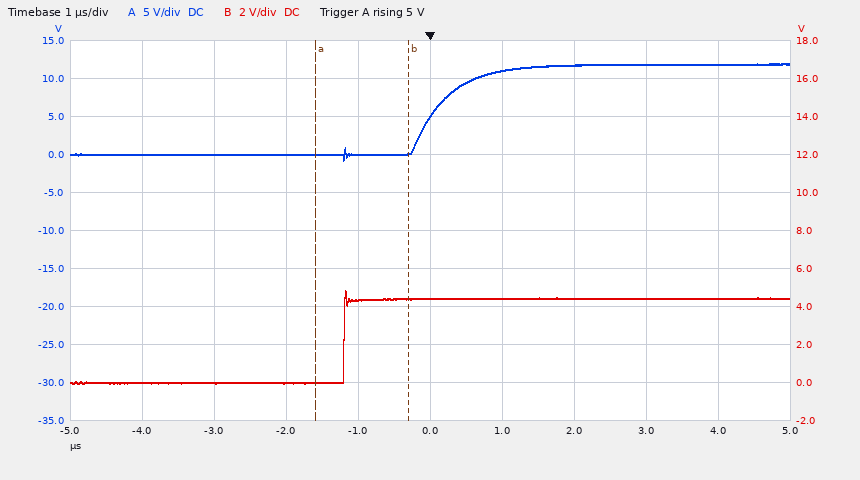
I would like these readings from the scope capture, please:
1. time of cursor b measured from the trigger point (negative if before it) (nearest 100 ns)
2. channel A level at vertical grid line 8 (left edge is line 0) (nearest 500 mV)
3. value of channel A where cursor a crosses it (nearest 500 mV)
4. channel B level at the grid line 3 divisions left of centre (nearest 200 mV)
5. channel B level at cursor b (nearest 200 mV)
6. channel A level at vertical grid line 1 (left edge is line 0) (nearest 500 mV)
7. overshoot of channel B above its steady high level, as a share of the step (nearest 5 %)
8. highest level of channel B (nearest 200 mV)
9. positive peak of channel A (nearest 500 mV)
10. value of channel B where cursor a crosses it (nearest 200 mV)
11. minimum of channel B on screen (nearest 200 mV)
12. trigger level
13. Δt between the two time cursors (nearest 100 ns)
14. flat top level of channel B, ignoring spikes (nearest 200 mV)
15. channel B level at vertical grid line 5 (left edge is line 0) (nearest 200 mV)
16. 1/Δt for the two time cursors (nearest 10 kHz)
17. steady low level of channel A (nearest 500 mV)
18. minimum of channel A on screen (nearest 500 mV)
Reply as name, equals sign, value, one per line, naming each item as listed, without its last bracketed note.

time of cursor b measured from the trigger point (negative if before it) = -300 ns
channel A level at vertical grid line 8 (left edge is line 0) = 12.0 V
value of channel A where cursor a crosses it = 0.0 V
channel B level at the grid line 3 divisions left of centre = 0.0 V
channel B level at cursor b = 4.4 V
channel A level at vertical grid line 1 (left edge is line 0) = 0.0 V
overshoot of channel B above its steady high level, as a share of the step = 10 %
highest level of channel B = 4.8 V
positive peak of channel A = 12.0 V
value of channel B where cursor a crosses it = 0.0 V
minimum of channel B on screen = 0.0 V
trigger level = 5 V
Δt between the two time cursors = 1.3 µs
flat top level of channel B, ignoring spikes = 4.4 V
channel B level at vertical grid line 5 (left edge is line 0) = 4.4 V
1/Δt for the two time cursors = 770 kHz
steady low level of channel A = 0.0 V
minimum of channel A on screen = -1.0 V
